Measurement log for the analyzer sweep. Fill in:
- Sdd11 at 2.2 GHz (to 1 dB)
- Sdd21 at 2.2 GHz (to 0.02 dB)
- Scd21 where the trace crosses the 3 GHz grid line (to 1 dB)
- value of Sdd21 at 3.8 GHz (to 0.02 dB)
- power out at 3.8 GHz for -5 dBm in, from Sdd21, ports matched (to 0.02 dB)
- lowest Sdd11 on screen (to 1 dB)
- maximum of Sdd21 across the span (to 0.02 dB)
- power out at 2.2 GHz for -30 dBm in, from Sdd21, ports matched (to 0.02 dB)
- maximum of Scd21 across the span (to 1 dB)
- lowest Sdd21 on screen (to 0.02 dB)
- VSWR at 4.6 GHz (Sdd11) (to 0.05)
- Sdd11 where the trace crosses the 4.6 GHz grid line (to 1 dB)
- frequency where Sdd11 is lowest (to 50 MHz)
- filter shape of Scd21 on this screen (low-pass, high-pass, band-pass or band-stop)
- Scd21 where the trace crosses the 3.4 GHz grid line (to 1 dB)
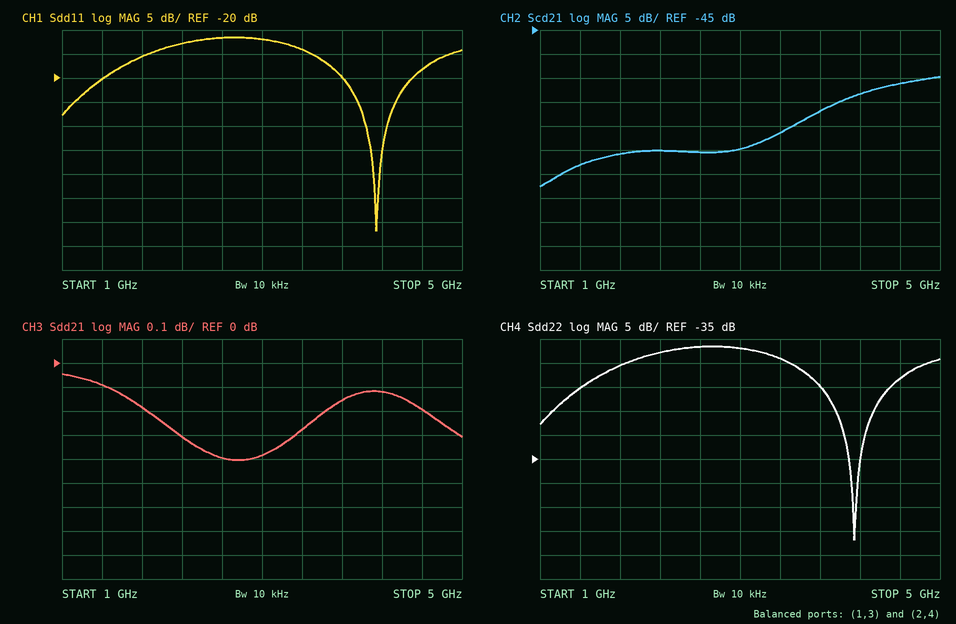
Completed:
-13 dB
-0.30 dB
-70 dB
-0.16 dB
-5.16 dBm
-52 dB
-0.04 dB
-30.30 dBm
-55 dB
-0.40 dB
1.30
-18 dB
4.15 GHz
high-pass
-66 dB
